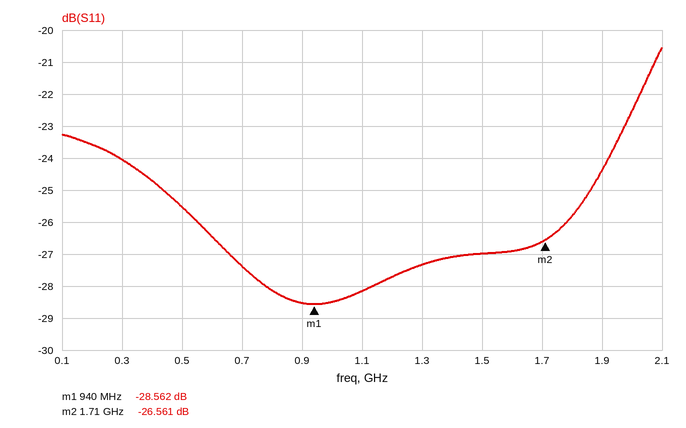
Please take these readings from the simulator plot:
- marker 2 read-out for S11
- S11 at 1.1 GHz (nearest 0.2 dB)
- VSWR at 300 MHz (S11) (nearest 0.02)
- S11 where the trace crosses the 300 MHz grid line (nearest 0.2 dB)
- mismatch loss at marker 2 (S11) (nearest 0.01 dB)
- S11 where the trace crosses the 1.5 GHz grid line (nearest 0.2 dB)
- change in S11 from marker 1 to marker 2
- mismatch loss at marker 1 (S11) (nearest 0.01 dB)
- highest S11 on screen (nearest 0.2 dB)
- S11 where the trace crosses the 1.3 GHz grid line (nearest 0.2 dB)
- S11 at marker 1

-26.561 dB
-28.2 dB
1.14
-24.0 dB
0.01 dB
-27.0 dB
2.001 dB
0.01 dB
-20.6 dB
-27.4 dB
-28.562 dB
